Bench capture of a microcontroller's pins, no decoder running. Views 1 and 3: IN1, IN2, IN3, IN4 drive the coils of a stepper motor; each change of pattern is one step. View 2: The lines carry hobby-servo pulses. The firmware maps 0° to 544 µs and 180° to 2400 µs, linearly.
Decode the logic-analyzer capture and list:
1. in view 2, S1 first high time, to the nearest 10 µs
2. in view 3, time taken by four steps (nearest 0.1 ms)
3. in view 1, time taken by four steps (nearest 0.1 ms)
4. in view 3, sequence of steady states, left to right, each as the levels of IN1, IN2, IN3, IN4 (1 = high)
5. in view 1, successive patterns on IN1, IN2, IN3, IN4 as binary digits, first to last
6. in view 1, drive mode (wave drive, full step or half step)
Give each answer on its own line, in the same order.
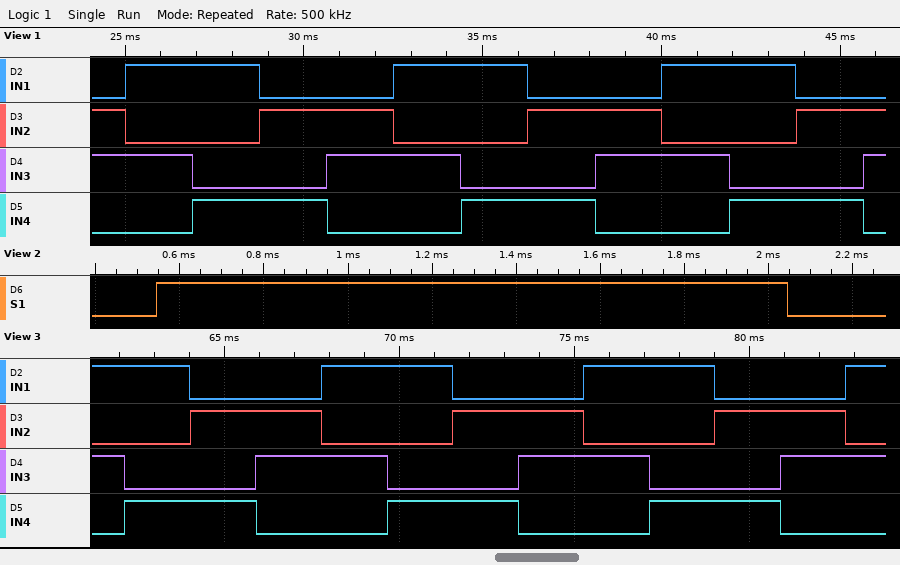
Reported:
1500 µs
7.5 ms
7.5 ms
1010 1001 0101 0110 1010 1001 0101 0110 1010 1001 0101 0110 1010
0110 1010 1001 0101 0110 1010 1001 0101 0110 1010 1001 0101 0110
full step
